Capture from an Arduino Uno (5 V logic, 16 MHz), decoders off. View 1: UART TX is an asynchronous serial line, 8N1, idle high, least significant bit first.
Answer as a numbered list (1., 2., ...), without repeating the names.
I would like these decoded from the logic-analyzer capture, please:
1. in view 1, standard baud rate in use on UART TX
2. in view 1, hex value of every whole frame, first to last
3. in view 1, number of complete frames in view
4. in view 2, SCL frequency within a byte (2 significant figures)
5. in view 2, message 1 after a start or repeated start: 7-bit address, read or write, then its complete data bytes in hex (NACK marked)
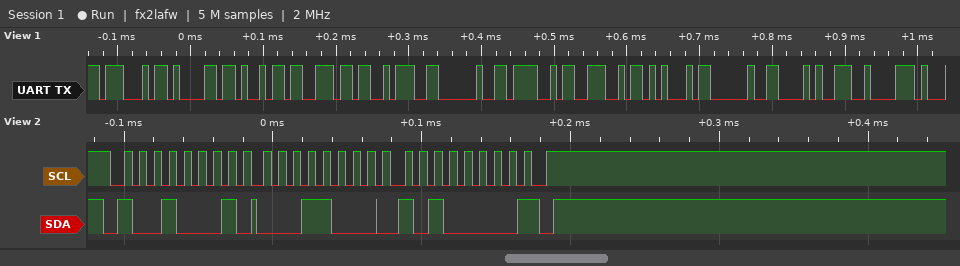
1. 115200 baud
2. 0x47 0x61 0x69 0x6E 0x3A 0x20 0x4F 0x4E 0x45 0x20 0x28 0xC2
3. 12
4. 100 kHz
5. 0x48 read: 18 A0 NACK
